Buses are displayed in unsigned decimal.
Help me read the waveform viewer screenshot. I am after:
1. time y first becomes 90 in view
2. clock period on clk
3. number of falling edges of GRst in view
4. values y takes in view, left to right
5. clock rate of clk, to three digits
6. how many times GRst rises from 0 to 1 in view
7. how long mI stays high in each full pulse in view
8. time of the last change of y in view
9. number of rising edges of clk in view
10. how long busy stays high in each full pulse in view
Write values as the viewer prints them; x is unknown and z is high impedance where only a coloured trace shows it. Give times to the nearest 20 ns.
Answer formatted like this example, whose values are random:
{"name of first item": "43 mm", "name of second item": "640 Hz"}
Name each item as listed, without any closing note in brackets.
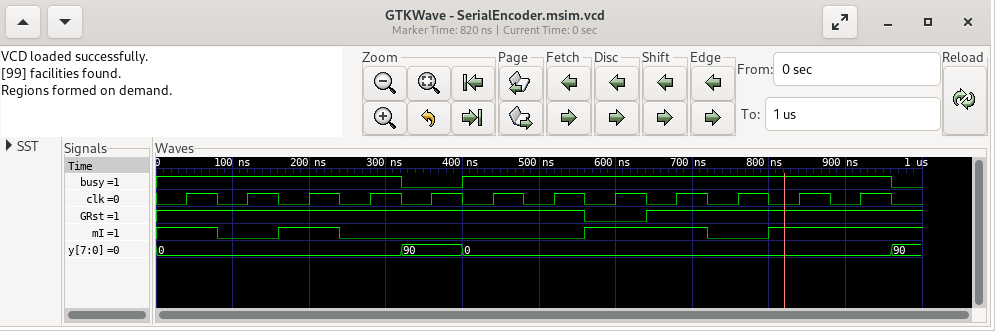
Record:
{"time y first becomes 90 in view": "320 ns", "clock period on clk": "80 ns", "number of falling edges of GRst in view": "1", "values y takes in view, left to right": "0, 90, 0, 90", "clock rate of clk, to three digits": "12.5 MHz", "how many times GRst rises from 0 to 1 in view": "1", "how long mI stays high in each full pulse in view": "80 ns, 160 ns", "time of the last change of y in view": "960 ns", "number of rising edges of clk in view": "12", "how long busy stays high in each full pulse in view": "560 ns"}
